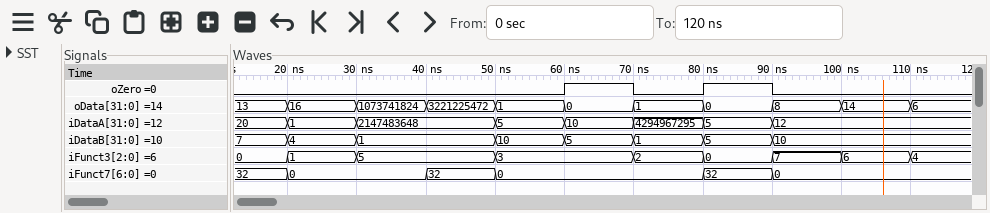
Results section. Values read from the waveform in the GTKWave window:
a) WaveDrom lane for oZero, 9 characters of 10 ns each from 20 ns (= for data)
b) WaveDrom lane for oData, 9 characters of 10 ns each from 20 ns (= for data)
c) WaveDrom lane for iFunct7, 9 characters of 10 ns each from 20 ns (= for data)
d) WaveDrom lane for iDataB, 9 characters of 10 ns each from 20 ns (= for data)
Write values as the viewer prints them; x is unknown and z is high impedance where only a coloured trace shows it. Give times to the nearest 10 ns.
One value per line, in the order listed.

{name: 'oZero', wave: '0...1010.'}
{name: 'oData', wave: '=========', data: '16 1073741824 3221225472 1 0 1 0 8 14'}
{name: 'iFunct7', wave: '=.==..==.', data: '0 32 0 32 0'}
{name: 'iDataB', wave: '==.=====.', data: '4 1 10 5 1 5 10'}
